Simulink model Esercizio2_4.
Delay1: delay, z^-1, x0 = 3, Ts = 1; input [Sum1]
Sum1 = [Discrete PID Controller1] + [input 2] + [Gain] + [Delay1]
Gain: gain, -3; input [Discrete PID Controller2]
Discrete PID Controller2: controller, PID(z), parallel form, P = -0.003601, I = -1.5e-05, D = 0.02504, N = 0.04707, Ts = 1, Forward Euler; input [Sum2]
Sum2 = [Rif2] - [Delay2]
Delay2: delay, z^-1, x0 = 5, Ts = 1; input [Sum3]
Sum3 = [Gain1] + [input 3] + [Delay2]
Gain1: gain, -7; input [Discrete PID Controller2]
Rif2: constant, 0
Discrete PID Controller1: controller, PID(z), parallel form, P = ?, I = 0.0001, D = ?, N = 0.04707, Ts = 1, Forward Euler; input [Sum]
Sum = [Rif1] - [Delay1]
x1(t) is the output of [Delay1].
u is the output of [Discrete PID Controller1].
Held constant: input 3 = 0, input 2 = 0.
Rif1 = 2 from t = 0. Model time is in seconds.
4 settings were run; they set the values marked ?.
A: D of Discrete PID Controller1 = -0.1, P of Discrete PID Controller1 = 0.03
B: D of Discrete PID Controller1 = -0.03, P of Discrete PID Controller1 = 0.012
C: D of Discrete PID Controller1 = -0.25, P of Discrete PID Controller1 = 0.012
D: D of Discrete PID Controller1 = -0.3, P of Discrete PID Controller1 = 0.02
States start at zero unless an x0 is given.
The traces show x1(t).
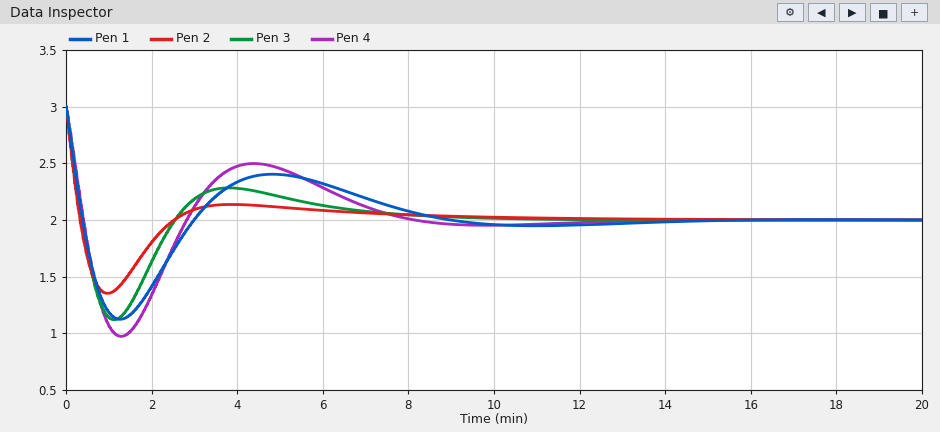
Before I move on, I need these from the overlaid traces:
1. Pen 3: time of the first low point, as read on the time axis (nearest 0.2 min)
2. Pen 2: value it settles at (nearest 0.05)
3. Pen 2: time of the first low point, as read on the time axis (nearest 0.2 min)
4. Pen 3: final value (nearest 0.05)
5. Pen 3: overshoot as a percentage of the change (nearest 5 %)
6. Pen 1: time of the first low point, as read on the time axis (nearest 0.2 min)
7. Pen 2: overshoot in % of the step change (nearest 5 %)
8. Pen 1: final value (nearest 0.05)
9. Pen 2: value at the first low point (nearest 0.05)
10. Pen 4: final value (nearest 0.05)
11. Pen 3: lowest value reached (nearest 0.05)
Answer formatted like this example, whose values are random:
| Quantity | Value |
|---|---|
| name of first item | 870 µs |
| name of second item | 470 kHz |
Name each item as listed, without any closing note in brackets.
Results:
| Quantity | Value |
|---|---|
| Pen 3: time of the first low point, as read on the time axis | 1.2 min |
| Pen 2: value it settles at | 2.00 |
| Pen 2: time of the first low point, as read on the time axis | 1.0 min |
| Pen 3: final value | 2.00 |
| Pen 3: overshoot as a percentage of the change | 90 % |
| Pen 1: time of the first low point, as read on the time axis | 1.2 min |
| Pen 2: overshoot in % of the step change | 65 % |
| Pen 1: final value | 2.00 |
| Pen 2: value at the first low point | 1.35 |
| Pen 4: final value | 2.00 |
| Pen 3: lowest value reached | 1.10 |
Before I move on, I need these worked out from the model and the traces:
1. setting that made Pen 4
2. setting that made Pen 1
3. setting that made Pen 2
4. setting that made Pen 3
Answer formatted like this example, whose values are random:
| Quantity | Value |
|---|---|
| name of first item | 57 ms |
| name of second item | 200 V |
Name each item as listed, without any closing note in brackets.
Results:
| Quantity | Value |
|---|---|
| setting that made Pen 4 | C |
| setting that made Pen 1 | B |
| setting that made Pen 2 | A |
| setting that made Pen 3 | D |
